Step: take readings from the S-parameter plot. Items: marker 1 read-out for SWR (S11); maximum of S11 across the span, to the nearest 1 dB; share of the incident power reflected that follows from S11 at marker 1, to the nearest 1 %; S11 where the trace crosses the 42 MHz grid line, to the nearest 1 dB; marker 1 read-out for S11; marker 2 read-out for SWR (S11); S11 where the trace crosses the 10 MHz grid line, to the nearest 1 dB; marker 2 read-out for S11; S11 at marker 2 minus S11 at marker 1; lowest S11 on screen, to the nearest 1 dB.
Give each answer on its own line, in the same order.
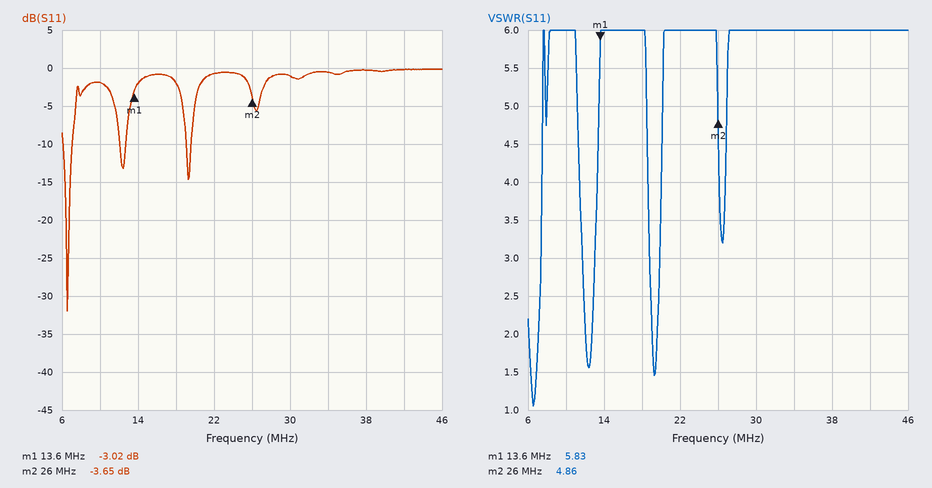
5.83
0 dB
50 %
0 dB
-3.02 dB
4.86
-2 dB
-3.65 dB
-0.63 dB
-32 dB
